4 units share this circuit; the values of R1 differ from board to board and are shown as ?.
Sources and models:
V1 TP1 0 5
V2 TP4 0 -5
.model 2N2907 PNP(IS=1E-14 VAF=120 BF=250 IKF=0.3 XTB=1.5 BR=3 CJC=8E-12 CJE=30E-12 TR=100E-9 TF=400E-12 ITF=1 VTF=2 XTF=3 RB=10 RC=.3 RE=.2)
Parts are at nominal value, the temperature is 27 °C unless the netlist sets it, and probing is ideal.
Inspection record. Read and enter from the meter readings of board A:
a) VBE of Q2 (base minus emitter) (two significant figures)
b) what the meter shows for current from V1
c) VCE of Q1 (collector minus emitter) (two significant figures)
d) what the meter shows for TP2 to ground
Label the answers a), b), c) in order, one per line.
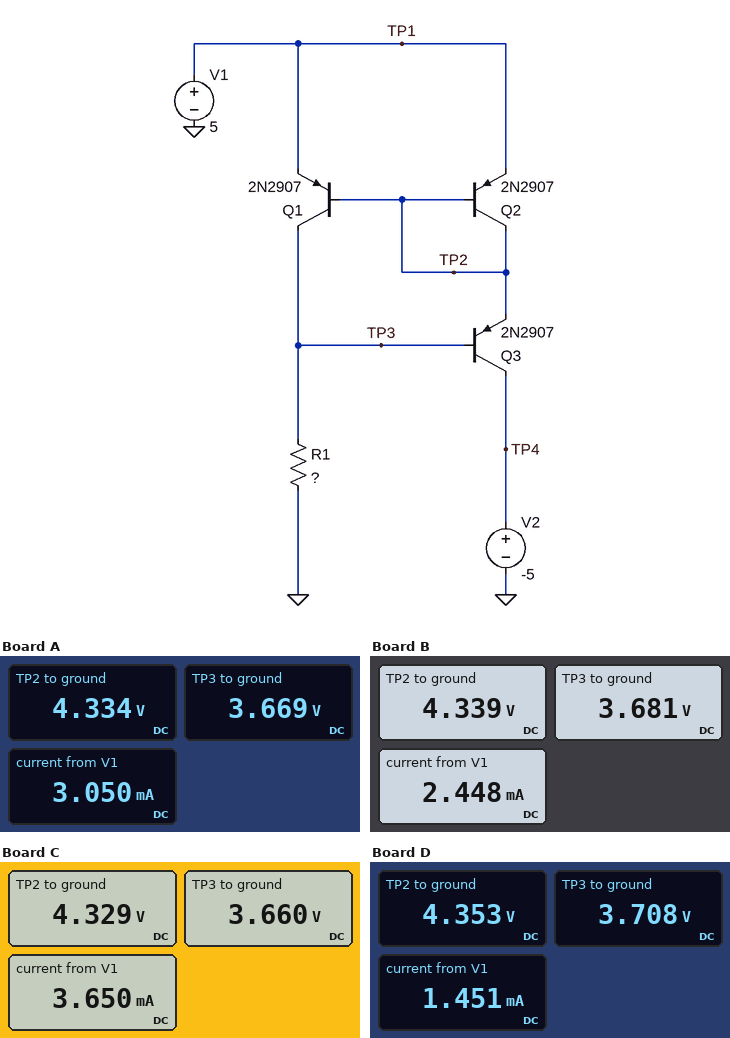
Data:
a) -670 mV
b) 3.050 mA
c) -1.3 V
d) 4.334 V
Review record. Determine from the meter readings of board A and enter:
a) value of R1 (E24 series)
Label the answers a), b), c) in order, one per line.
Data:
a) 2.4 kΩ
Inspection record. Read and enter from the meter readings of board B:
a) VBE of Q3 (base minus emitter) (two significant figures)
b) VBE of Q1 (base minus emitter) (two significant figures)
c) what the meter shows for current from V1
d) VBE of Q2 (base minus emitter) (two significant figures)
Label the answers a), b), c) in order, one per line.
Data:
a) -660 mV
b) -660 mV
c) 2.448 mA
d) -660 mV
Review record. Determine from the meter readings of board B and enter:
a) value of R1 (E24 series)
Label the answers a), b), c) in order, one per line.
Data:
a) 3 kΩ
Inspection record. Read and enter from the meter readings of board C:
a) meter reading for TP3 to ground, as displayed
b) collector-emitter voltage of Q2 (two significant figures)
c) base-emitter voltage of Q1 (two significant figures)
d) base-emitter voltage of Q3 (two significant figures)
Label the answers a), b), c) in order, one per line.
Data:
a) 3.660 V
b) -670 mV
c) -670 mV
d) -670 mV
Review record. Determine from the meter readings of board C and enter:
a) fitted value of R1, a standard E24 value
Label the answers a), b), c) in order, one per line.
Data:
a) 2 kΩ
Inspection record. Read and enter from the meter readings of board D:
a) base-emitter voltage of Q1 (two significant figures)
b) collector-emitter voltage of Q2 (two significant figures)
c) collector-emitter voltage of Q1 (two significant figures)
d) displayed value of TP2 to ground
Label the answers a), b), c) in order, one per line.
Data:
a) -650 mV
b) -650 mV
c) -1.3 V
d) 4.353 V
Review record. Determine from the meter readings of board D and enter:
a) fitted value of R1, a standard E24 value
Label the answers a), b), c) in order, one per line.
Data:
a) 5.1 kΩ
